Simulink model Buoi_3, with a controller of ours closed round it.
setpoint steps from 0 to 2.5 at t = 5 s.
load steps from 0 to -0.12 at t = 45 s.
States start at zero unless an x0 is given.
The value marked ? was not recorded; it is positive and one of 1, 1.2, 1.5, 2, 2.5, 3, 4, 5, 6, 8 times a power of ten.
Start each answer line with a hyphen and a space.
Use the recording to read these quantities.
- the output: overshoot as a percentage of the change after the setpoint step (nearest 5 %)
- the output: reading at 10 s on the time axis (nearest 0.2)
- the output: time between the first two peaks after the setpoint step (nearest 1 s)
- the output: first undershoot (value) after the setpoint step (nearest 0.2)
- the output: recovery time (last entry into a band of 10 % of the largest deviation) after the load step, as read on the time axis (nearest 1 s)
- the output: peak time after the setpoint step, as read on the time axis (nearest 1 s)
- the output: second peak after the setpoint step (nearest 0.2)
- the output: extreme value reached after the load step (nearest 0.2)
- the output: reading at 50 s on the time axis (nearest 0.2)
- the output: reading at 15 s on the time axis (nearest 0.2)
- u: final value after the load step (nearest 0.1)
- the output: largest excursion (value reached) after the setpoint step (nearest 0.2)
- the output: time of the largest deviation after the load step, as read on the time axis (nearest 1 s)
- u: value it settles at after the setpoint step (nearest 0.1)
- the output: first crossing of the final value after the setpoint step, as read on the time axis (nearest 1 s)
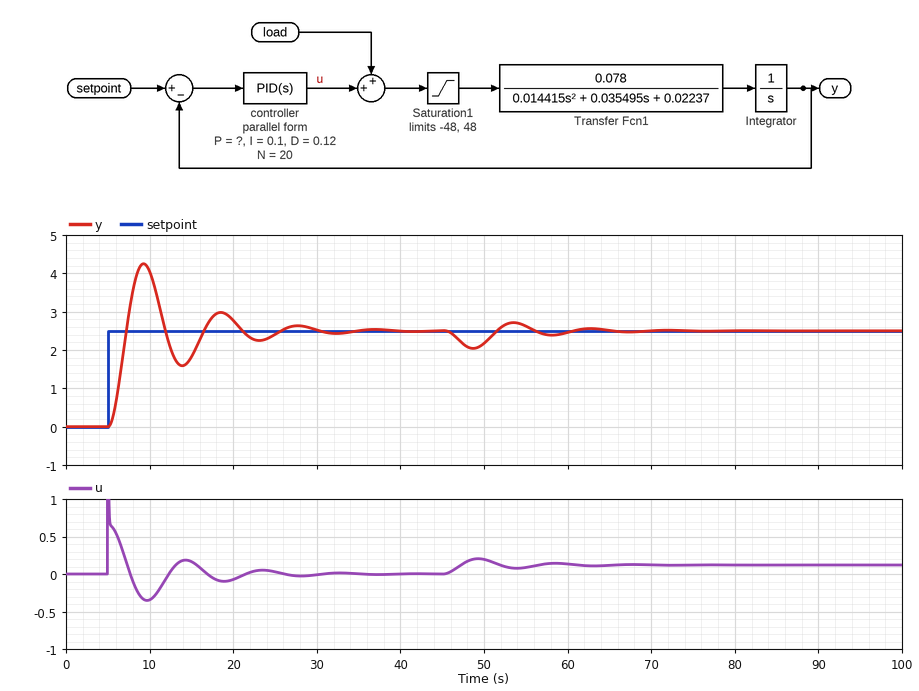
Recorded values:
- 70 %
- 4.0
- 9 s
- 1.6
- 64 s
- 9 s
- 3.0
- 2.0
- 2.2
- 1.8
- 0.1
- 4.2
- 49 s
- 0.0
- 7 s
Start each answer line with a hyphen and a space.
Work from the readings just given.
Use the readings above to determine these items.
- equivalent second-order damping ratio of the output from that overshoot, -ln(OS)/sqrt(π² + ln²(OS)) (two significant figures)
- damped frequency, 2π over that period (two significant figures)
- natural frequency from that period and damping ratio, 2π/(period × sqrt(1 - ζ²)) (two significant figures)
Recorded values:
- 0.11
- 0.70 rad/s
- 0.70 rad/s
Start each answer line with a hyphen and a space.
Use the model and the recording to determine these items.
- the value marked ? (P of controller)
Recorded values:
- 0.25
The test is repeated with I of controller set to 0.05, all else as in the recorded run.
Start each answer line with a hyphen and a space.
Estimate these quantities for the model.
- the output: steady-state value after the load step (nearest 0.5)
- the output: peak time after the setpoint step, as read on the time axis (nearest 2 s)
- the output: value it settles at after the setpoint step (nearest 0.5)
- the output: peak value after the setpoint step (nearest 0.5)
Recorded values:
- 2.5
- 10 s
- 2.5
- 3.5
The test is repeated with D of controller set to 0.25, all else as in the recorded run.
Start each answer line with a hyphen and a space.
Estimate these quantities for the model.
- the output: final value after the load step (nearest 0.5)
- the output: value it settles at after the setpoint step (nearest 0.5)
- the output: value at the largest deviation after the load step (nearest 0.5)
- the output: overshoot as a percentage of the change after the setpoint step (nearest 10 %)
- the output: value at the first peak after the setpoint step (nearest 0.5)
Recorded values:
- 2.5
- 2.5
- 2.0
- 40 %
- 3.5
